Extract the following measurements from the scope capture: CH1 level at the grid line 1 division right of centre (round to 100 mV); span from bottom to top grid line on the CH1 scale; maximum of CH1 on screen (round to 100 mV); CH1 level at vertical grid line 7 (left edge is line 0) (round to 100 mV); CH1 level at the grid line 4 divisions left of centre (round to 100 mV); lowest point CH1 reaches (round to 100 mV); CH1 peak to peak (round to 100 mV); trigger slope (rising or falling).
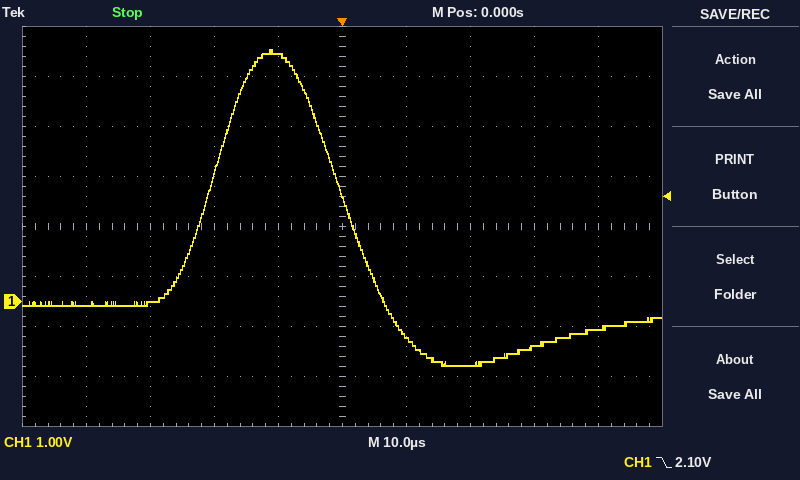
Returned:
-700 mV
8 V
5.0 V
-1.3 V
-100 mV
-1.3 V
6.3 V
falling
